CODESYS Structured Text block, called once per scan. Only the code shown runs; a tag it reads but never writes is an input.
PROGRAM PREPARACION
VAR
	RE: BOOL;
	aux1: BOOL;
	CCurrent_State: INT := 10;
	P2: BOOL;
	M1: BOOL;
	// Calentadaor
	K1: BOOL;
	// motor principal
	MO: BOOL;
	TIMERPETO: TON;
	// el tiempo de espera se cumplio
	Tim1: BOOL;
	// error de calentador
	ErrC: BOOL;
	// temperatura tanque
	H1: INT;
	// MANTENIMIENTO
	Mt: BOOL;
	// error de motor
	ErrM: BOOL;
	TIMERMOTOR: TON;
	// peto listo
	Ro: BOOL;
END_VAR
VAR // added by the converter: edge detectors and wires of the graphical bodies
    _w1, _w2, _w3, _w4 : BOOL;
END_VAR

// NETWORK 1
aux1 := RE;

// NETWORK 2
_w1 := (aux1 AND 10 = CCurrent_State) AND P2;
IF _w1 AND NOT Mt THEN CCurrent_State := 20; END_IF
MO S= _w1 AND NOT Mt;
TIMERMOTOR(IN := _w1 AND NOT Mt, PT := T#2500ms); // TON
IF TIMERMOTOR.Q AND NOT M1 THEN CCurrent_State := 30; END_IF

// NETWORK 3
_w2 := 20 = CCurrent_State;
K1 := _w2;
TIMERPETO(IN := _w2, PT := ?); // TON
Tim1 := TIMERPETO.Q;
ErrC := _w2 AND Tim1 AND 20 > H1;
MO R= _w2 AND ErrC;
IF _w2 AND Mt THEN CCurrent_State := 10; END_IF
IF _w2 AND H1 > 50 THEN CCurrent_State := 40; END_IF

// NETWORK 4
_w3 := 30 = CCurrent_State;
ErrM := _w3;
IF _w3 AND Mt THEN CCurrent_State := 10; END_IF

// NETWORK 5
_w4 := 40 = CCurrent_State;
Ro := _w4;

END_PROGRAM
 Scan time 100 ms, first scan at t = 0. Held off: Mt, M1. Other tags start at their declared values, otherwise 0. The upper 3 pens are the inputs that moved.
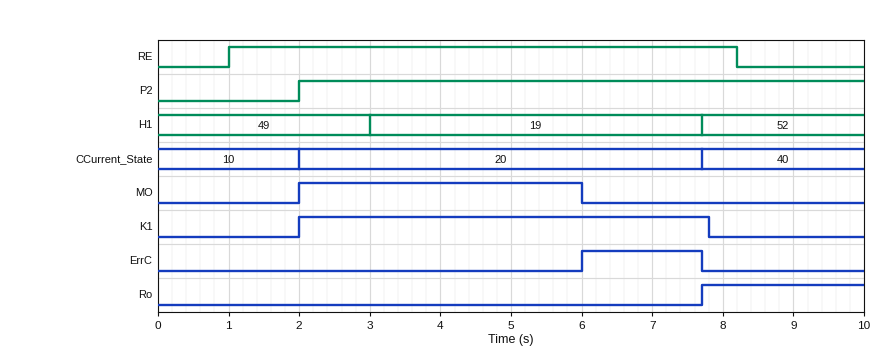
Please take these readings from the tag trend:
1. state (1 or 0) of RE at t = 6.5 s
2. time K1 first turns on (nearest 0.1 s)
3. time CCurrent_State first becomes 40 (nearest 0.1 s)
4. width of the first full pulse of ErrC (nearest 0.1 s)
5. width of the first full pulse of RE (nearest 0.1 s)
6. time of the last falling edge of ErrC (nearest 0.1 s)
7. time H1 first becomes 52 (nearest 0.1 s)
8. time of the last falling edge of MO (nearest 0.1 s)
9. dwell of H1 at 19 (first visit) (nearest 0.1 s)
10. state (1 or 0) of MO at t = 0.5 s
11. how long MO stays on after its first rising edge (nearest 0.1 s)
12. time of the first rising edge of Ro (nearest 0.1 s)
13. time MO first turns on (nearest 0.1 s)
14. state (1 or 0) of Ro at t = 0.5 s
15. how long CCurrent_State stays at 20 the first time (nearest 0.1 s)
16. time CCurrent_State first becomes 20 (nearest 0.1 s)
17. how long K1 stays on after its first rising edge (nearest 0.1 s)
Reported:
1
2.0 s
7.7 s
1.7 s
7.2 s
7.7 s
7.7 s
6.0 s
4.7 s
0
4.0 s
7.7 s
2.0 s
0
5.7 s
2.0 s
5.8 s
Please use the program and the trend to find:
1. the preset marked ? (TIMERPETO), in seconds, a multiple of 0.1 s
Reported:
4.0 s
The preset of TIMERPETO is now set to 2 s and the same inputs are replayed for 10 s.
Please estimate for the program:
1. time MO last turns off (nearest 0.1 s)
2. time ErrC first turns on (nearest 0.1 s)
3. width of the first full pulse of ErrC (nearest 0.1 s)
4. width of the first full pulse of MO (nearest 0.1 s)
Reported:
4.0 s
4.0 s
3.7 s
2.0 s
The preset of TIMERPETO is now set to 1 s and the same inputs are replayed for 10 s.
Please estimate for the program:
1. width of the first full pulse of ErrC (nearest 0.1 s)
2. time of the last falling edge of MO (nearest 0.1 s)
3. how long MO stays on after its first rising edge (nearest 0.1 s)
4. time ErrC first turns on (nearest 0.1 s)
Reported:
4.7 s
3.0 s
1.0 s
3.0 s
